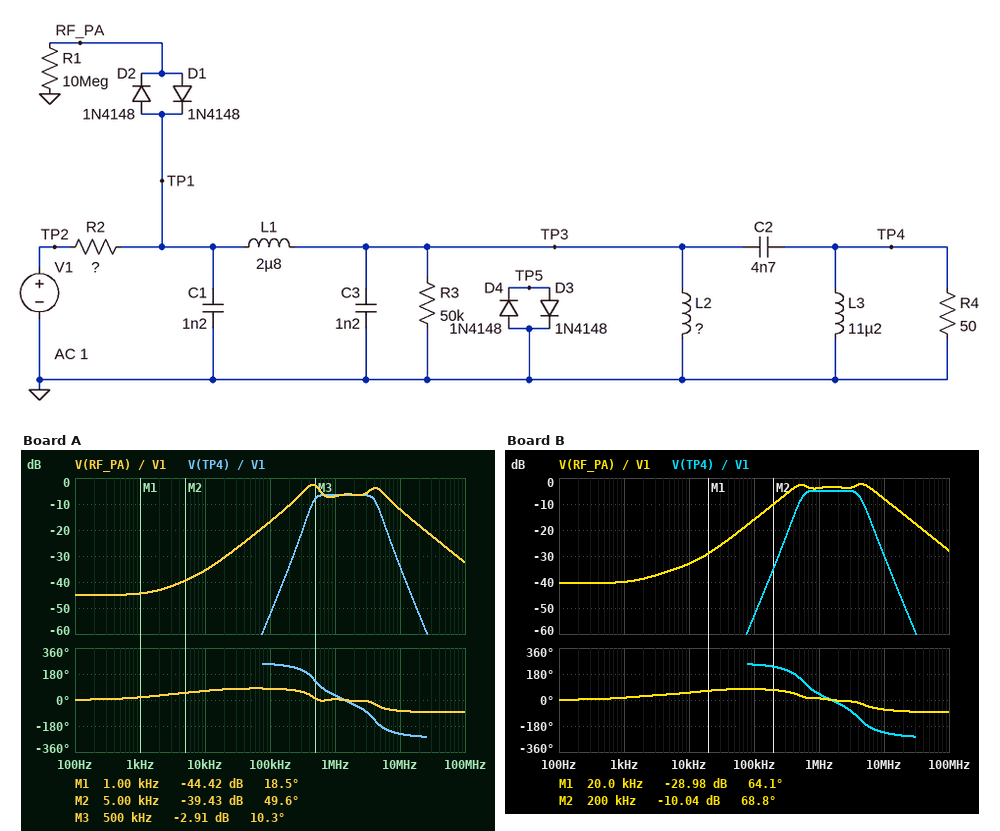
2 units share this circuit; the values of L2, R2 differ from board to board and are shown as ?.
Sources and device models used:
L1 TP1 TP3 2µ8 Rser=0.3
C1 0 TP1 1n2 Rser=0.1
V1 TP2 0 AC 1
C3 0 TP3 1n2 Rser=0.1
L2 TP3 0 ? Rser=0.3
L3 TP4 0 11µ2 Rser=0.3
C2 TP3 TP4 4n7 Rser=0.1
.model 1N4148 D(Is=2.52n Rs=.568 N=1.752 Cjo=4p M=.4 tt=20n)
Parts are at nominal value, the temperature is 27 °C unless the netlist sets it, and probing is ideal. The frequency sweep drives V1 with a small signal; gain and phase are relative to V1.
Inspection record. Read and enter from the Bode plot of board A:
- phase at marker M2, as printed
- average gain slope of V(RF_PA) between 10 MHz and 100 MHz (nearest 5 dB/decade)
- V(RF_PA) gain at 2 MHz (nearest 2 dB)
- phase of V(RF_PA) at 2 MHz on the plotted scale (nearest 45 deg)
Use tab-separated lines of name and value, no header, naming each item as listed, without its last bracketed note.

phase at marker M2, as printed	49.6 deg
average gain slope of V(RF_PA) between 10 MHz and 100 MHz	-20 dB/decade
V(RF_PA) gain at 2 MHz	-6 dB
phase of V(RF_PA) at 2 MHz on the plotted scale	0 deg
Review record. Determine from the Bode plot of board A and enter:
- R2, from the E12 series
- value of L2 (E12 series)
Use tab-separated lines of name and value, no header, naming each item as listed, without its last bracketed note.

R2, from the E12 series	56 Ω
value of L2	10 µH
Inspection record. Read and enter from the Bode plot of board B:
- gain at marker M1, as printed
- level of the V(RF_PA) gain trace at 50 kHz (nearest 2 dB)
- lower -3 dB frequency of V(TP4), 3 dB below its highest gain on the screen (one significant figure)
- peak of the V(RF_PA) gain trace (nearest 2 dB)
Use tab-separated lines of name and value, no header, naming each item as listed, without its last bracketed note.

gain at marker M1, as printed	-28.98 dB
level of the V(RF_PA) gain trace at 50 kHz	-22 dB
lower -3 dB frequency of V(TP4), 3 dB below its highest gain on the screen	500 kHz
peak of the V(RF_PA) gain trace	-2 dB
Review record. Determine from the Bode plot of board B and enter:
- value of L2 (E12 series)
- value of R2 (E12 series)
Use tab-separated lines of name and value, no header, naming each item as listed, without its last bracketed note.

value of L2	5.6 µH
value of R2	33 Ω
